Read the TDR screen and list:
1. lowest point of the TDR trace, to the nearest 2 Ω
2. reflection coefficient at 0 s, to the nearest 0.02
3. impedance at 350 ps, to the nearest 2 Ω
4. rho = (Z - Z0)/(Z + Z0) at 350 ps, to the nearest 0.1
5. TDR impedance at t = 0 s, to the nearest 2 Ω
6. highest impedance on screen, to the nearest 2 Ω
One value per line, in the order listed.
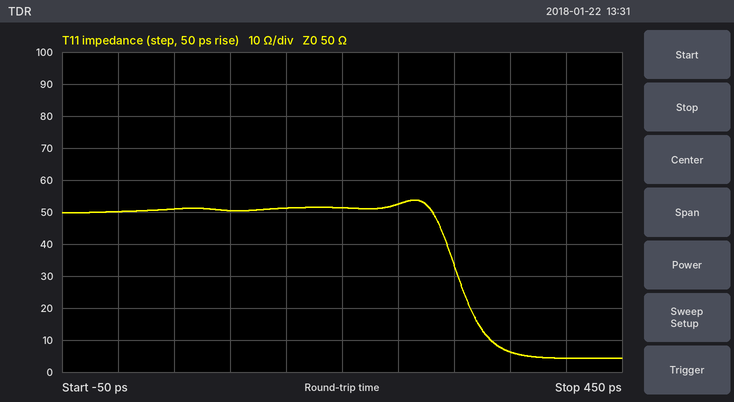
4 Ω
0.00
6 Ω
-0.8
50 Ω
54 Ω
